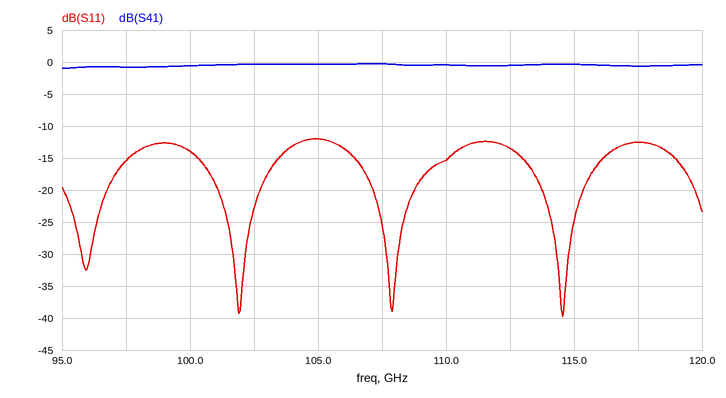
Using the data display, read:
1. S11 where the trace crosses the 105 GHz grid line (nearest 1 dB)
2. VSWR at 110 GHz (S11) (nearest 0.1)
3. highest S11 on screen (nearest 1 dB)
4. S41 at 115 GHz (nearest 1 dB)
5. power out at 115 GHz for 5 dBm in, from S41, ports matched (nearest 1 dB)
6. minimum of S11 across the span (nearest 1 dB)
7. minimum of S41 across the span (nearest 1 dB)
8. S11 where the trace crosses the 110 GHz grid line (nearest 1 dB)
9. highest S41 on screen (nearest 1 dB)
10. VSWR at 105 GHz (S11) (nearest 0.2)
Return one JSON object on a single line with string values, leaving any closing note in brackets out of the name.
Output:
{"S11 where the trace crosses the 105 GHz grid line": "-12 dB", "VSWR at 110 GHz (S11)": "1.4", "highest S11 on screen": "-12 dB", "S41 at 115 GHz": "0 dB", "power out at 115 GHz for 5 dBm in, from S41, ports matched": "5 dBm", "minimum of S11 across the span": "-40 dB", "minimum of S41 across the span": "-1 dB", "S11 where the trace crosses the 110 GHz grid line": "-15 dB", "highest S41 on screen": "0 dB", "VSWR at 105 GHz (S11)": "1.6"}
